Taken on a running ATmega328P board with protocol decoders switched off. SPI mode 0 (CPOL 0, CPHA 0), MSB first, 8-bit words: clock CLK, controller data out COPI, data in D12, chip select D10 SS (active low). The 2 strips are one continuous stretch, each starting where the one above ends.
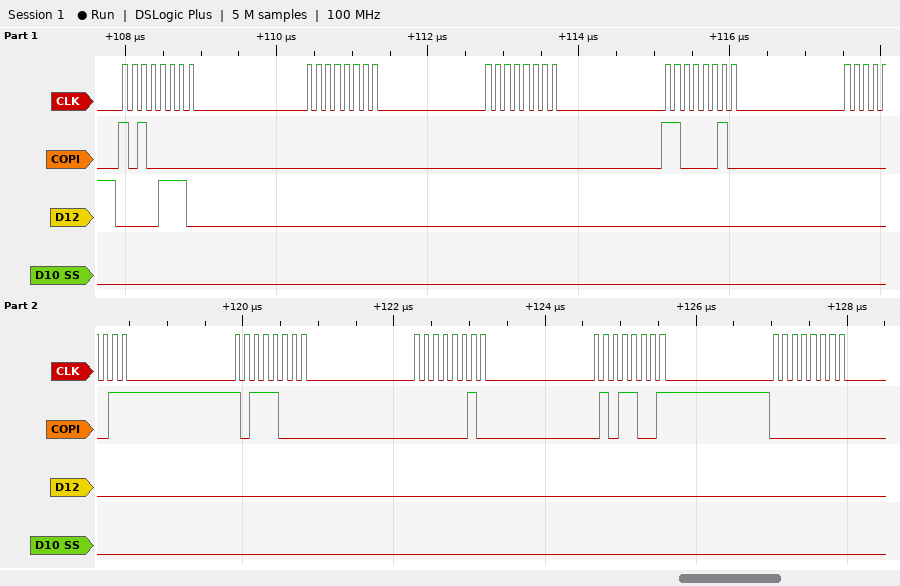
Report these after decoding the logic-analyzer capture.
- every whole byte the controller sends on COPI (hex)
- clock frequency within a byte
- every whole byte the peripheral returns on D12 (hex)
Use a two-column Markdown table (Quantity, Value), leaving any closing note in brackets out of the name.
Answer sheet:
| Quantity | Value |
|---|---|
| every whole byte the controller sends on COPI | A0 00 00 C2 03 B8 02 59 00 |
| clock frequency within a byte | 8 MHz |
| every whole byte the peripheral returns on D12 | 0E 00 00 00 00 00 00 00 00 |
